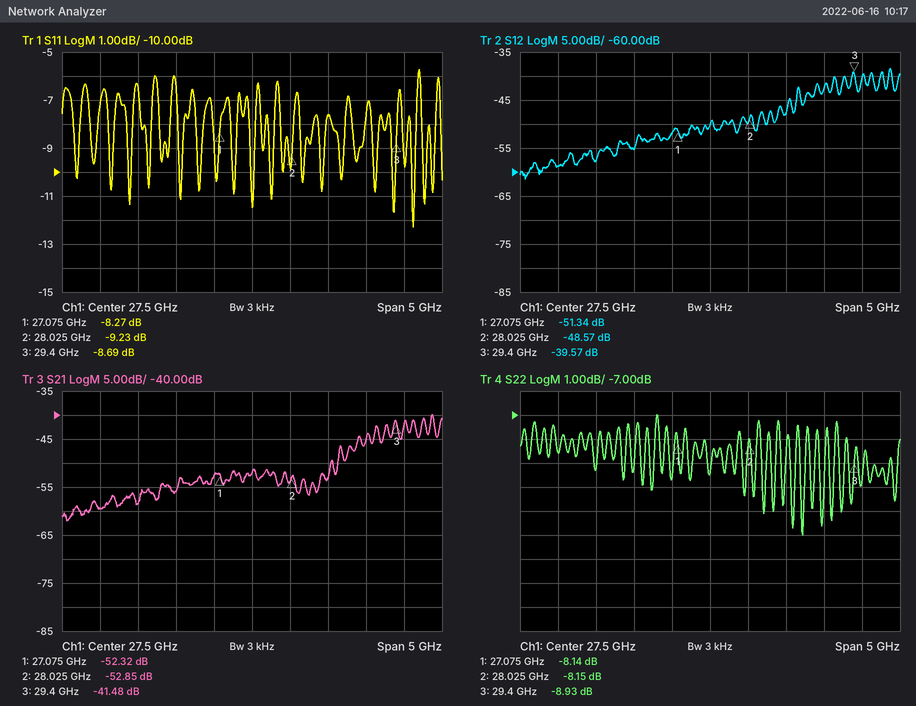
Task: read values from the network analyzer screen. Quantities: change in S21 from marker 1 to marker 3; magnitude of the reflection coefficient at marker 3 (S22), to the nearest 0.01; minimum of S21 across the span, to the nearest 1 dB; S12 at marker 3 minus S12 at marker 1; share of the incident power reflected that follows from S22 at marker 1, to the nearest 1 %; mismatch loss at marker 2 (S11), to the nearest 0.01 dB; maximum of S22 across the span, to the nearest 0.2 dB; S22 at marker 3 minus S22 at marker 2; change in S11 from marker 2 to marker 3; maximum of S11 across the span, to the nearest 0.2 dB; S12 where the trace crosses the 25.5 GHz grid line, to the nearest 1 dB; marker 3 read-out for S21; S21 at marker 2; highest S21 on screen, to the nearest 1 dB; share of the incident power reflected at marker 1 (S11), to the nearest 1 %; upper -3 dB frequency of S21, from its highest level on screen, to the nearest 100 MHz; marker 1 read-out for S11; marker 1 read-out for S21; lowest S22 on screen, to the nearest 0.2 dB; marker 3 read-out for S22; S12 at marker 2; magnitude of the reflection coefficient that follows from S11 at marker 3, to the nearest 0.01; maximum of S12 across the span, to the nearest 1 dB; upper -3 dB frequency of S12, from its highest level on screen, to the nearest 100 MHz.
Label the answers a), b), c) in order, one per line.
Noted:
a) 10.84 dB
b) 0.36
c) -62 dB
d) 11.77 dB
e) 15 %
f) 0.55 dB
g) -7.0 dB
h) -0.78 dB
i) 0.54 dB
j) -5.8 dB
k) -59 dB
l) -41.48 dB
m) -52.85 dB
n) -40 dB
o) 15 %
p) 29.9 GHz
q) -8.27 dB
r) -52.32 dB
s) -12.0 dB
t) -8.93 dB
u) -48.57 dB
v) 0.37
w) -38 dB
x) 29.9 GHz
